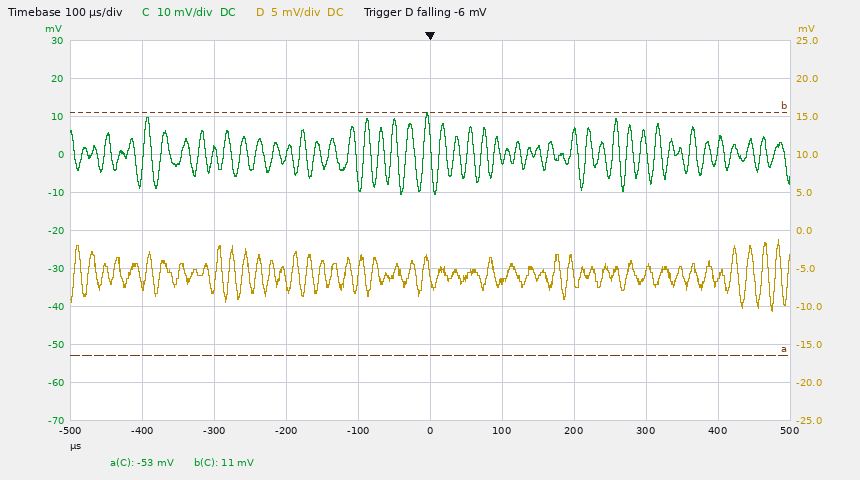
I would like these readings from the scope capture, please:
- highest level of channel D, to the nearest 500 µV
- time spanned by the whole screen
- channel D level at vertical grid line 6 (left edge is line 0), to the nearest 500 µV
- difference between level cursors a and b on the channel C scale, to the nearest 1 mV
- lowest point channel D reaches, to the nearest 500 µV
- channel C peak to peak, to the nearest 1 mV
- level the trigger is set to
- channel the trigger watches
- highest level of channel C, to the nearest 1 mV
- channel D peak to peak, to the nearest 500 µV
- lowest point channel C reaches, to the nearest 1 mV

-1.0 mV
1 ms
-6.5 mV
64 mV
-10.5 mV
22 mV
-6 mV
channel D
11 mV
9.5 mV
-11 mV
